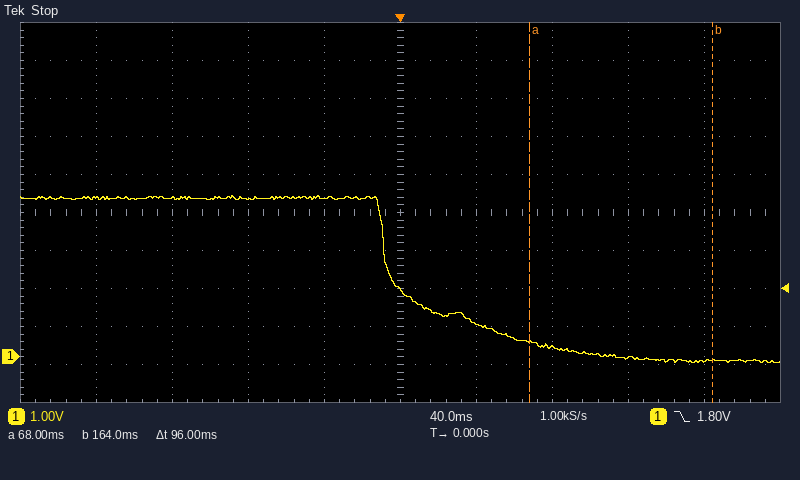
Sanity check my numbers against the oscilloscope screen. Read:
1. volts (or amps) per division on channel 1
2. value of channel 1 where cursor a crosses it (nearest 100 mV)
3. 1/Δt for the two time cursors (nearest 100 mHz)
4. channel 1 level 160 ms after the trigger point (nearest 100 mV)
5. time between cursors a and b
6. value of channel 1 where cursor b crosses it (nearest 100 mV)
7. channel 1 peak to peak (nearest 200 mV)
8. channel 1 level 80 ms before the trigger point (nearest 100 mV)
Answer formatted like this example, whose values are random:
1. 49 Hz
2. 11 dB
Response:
1. 1 V
2. 400 mV
3. 10.4 Hz
4. -100 mV
5. 96 ms
6. -100 mV
7. 4.4 V
8. 4.2 V
